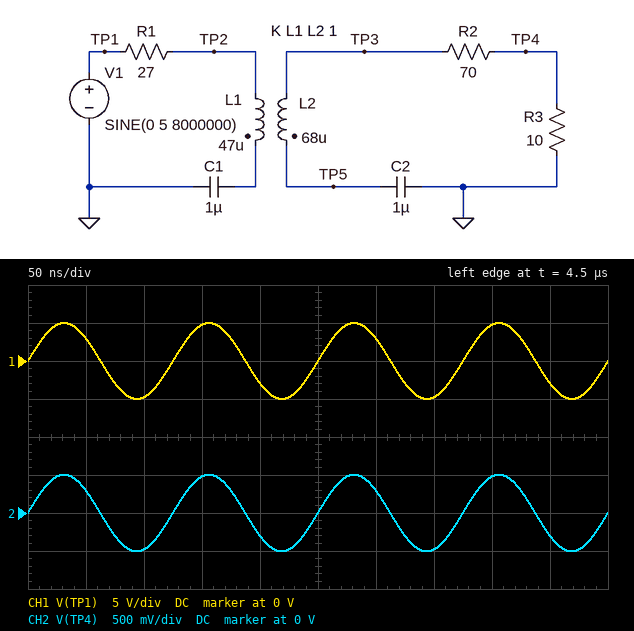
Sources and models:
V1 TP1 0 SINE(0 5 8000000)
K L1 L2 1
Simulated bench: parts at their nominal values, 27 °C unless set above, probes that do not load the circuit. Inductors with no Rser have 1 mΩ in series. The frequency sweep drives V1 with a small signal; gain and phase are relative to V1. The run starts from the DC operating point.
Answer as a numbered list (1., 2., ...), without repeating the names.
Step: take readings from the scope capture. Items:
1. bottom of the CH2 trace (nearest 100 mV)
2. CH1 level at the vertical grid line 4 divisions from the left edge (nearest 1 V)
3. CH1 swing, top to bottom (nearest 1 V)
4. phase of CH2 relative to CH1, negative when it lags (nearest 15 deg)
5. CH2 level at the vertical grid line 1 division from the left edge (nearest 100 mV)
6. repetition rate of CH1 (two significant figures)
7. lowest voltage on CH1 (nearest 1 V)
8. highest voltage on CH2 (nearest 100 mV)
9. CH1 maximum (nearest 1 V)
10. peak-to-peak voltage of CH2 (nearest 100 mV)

1. -500 mV
2. -3 V
3. 10 V
4. 0 deg
5. 300 mV
6. 8.0 MHz
7. -5 V
8. 500 mV
9. 5 V
10. 1.0 V
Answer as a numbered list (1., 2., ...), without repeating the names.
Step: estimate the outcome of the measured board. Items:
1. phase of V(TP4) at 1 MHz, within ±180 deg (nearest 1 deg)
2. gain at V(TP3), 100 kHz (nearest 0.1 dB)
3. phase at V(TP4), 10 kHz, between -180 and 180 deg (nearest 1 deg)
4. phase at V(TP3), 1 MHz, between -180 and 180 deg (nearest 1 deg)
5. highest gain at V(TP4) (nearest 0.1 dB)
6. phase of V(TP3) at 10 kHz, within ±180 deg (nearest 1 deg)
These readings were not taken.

1. 4 deg
2. -3.1 dB
3. 124 deg
4. 4 deg
5. -19.9 dB
6. 124 deg
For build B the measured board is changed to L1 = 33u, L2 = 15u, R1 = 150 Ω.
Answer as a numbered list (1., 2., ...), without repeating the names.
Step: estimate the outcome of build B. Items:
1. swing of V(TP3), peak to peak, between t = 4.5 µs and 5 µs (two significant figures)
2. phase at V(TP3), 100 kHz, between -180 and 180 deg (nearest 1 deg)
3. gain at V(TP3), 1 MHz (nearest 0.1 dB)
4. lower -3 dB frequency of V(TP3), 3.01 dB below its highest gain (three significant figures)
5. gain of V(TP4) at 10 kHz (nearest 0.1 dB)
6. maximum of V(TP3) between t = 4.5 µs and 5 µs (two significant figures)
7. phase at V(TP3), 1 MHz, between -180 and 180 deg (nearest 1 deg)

1. 3.6 V
2. 77 deg
3. -9.4 dB
4. 389 kHz
5. -58.9 dB
6. 1.8 V
7. 21 deg
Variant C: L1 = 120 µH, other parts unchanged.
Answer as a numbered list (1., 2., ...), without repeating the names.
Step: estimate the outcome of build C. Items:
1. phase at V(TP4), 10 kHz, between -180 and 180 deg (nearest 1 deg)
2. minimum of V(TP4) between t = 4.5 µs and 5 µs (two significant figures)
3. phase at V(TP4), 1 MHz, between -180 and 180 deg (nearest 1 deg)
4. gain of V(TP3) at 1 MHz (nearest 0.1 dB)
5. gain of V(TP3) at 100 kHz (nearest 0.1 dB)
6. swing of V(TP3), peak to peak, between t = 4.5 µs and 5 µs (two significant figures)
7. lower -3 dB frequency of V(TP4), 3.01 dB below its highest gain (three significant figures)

1. 115 deg
2. -400 mV
3. 2 deg
4. -4.0 dB
5. -4.2 dB
6. 6.3 V
7. 25.4 kHz
